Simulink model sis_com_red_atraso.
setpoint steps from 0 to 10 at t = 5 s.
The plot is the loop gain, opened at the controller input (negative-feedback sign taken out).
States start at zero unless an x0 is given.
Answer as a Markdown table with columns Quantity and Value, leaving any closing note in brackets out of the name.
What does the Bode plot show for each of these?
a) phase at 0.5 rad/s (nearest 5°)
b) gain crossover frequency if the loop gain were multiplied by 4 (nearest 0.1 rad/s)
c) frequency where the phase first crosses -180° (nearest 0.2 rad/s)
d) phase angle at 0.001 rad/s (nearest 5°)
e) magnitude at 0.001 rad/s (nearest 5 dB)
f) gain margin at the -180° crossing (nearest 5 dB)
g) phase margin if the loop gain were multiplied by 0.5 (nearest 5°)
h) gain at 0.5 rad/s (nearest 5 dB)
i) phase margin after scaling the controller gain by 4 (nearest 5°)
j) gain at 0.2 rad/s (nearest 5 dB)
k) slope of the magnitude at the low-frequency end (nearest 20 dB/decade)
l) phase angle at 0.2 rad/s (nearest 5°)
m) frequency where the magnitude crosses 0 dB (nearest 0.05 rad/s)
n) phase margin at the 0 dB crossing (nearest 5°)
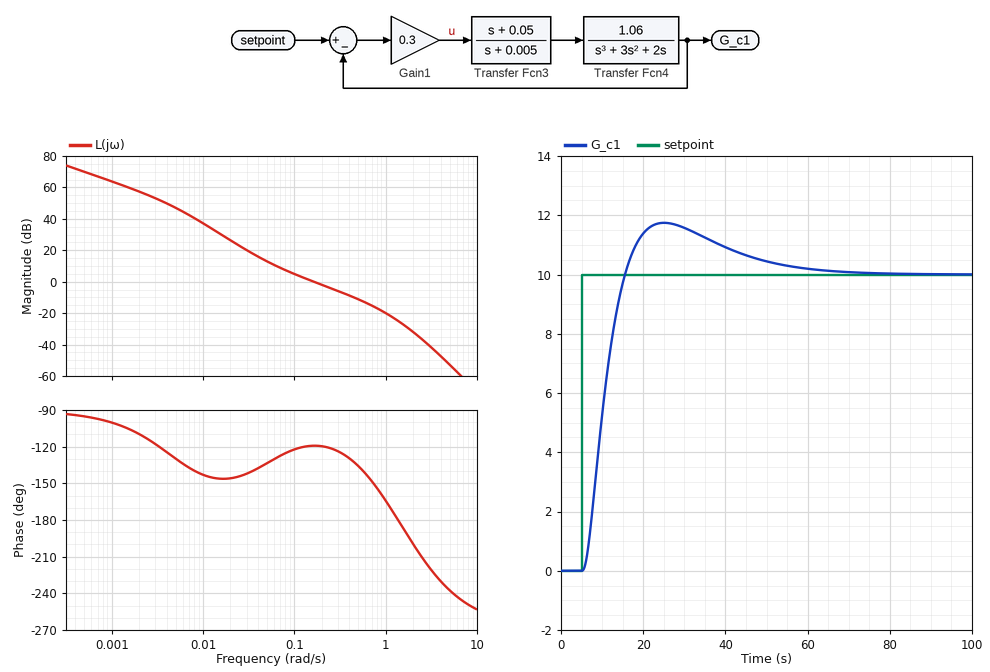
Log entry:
| Quantity | Value |
|---|---|
| phase at 0.5 rad/s | -135° |
| gain crossover frequency if the loop gain were multiplied by 4 | 0.5 rad/s |
| frequency where the phase first crosses -180° | 1.4 rad/s |
| phase angle at 0.001 rad/s | -100° |
| magnitude at 0.001 rad/s | 65 dB |
| gain margin at the -180° crossing | 25 dB |
| phase margin if the loop gain were multiplied by 0.5 | 55° |
| gain at 0.5 rad/s | -10 dB |
| phase margin after scaling the controller gain by 4 | 40° |
| gain at 0.2 rad/s | 0 dB |
| slope of the magnitude at the low-frequency end | -20 dB/decade |
| phase angle at 0.2 rad/s | -120° |
| frequency where the magnitude crosses 0 dB | 0.15 rad/s |
| phase margin at the 0 dB crossing | 60° |
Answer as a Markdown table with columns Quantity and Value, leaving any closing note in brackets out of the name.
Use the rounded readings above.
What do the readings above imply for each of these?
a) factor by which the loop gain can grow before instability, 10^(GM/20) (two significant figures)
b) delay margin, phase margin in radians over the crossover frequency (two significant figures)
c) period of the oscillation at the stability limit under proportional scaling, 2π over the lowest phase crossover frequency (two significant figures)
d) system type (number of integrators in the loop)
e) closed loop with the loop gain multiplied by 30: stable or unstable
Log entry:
| Quantity | Value |
|---|---|
| factor by which the loop gain can grow before instability, 10^(GM/20) | 18 |
| delay margin, phase margin in radians over the crossover frequency | 7.0 s |
| period of the oscillation at the stability limit under proportional scaling, 2π over the lowest phase crossover frequency | 4.5 s |
| system type | 1 |
| closed loop with the loop gain multiplied by 30: stable or unstable | unstable |
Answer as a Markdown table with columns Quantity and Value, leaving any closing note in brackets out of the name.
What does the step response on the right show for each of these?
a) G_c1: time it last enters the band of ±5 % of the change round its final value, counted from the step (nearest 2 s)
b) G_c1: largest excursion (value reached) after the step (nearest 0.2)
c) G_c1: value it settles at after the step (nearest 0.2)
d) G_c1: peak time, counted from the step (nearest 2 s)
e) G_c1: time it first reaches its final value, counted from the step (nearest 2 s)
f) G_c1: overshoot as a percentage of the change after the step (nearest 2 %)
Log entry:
| Quantity | Value |
|---|---|
| G_c1: time it last enters the band of ±5 % of the change round its final value, counted from the step | 44 s |
| G_c1: largest excursion (value reached) after the step | 11.8 |
| G_c1: value it settles at after the step | 10.0 |
| G_c1: peak time, counted from the step | 20 s |
| G_c1: time it first reaches its final value, counted from the step | 10 s |
| G_c1: overshoot as a percentage of the change after the step | 18 % |
